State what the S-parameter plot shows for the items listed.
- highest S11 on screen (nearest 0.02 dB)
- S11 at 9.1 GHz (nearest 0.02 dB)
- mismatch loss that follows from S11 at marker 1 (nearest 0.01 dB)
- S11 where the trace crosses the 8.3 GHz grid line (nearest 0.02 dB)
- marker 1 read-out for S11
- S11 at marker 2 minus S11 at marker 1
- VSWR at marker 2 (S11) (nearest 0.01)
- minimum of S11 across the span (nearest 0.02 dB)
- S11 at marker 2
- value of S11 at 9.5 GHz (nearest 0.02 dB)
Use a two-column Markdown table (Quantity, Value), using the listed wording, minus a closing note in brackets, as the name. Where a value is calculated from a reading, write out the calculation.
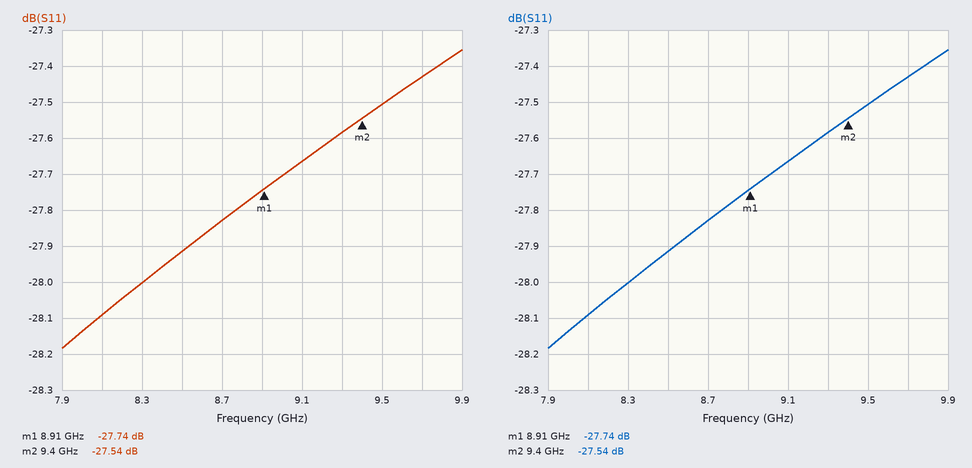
| Quantity | Value |
|---|---|
| highest S11 on screen | -27.36 dB |
| S11 at 9.1 GHz | -27.66 dB |
| mismatch loss that follows from S11 at marker 1 | −10 log10(1 − 10^(-27.74/10)) ≈ 0.01 dB |
| S11 where the trace crosses the 8.3 GHz grid line | -28.00 dB |
| marker 1 read-out for S11 | -27.74 dB |
| S11 at marker 2 minus S11 at marker 1 | -27.54 − (-27.74) = 0.20 dB |
| VSWR at marker 2 (S11) | (1 + 0.0420)/(1 − 0.0420) ≈ 1.09 |
| minimum of S11 across the span | -28.18 dB |
| S11 at marker 2 | -27.54 dB |
| value of S11 at 9.5 GHz | -27.50 dB |
